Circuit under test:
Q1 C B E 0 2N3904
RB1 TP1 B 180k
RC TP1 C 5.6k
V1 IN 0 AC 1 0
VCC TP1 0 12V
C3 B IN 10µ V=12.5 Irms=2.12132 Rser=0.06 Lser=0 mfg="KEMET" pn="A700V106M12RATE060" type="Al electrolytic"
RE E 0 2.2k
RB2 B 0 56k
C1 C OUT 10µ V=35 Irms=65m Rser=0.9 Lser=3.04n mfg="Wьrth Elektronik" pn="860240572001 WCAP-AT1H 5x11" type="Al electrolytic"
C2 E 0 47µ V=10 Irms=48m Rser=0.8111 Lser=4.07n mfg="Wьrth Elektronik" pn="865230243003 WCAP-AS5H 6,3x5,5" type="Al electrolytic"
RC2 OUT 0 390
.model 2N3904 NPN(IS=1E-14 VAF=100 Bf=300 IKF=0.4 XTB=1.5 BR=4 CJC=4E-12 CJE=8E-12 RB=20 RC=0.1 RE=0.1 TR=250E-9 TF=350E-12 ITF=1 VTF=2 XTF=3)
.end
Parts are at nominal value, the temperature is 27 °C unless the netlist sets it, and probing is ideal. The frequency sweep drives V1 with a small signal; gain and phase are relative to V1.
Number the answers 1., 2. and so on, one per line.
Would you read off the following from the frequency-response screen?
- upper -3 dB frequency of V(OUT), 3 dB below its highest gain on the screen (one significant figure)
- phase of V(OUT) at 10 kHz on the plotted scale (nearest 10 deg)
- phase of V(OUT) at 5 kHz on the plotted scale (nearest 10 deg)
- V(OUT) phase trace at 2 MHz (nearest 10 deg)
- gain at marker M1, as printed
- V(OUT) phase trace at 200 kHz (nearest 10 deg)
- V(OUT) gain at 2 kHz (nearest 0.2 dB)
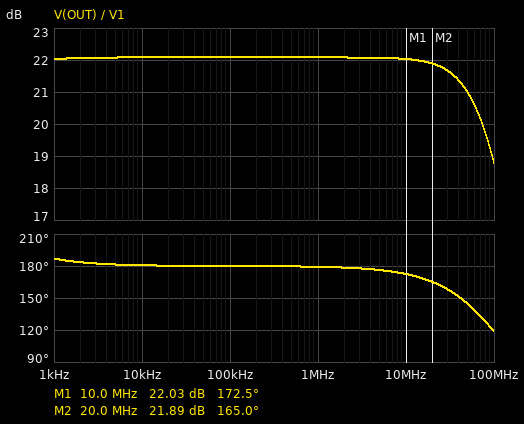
1. 90 MHz
2. 180 deg
3. 180 deg
4. 180 deg
5. 22.03 dB
6. 180 deg
7. 22.0 dB
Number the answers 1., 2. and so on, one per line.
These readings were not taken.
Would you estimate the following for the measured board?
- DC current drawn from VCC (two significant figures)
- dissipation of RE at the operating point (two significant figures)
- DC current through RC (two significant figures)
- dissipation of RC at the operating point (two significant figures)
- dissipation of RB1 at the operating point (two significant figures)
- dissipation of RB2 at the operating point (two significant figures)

1. 990 µA
2. 1.9 mW
3. 940 µA
4. 4.9 mW
5. 480 µW
6. 130 µW
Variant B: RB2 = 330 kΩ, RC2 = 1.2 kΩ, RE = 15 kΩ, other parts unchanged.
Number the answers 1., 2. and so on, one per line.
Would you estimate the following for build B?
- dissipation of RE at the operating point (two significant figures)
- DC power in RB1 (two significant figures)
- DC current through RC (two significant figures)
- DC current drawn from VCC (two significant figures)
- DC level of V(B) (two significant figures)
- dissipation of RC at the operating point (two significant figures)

1. 3.2 mW
2. 110 µW
3. 460 µA
4. 490 µA
5. 7.6 V
6. 1.2 mW
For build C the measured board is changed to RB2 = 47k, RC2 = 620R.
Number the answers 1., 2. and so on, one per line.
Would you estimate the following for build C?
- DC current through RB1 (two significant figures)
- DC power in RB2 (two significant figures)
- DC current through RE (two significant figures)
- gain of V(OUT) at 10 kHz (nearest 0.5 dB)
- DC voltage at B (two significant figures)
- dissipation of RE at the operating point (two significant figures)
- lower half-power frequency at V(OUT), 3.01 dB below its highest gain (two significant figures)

1. 53 µA
2. 120 µW
3. 790 µA
4. 24.5 dB
5. 2.4 V
6. 1.4 mW
7. 100 Hz
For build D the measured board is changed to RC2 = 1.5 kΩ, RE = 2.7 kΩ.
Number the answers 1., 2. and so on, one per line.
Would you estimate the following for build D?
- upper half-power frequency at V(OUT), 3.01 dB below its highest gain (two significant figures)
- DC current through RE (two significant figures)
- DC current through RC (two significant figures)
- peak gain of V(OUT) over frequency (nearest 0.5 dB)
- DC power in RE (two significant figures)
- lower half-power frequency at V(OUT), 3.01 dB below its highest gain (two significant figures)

1. 39 MHz
2. 780 µA
3. 770 µA
4. 30.5 dB
5. 1.6 mW
6. 100 Hz
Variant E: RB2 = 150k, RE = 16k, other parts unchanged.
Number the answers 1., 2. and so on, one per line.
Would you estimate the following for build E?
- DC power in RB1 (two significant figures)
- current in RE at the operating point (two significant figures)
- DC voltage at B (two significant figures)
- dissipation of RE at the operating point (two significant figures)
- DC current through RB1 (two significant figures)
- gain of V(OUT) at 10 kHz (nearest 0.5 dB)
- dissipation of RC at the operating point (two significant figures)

1. 240 µW
2. 300 µA
3. 5.4 V
4. 1.4 mW
5. 37 µA
6. 12.5 dB
7. 490 µW
